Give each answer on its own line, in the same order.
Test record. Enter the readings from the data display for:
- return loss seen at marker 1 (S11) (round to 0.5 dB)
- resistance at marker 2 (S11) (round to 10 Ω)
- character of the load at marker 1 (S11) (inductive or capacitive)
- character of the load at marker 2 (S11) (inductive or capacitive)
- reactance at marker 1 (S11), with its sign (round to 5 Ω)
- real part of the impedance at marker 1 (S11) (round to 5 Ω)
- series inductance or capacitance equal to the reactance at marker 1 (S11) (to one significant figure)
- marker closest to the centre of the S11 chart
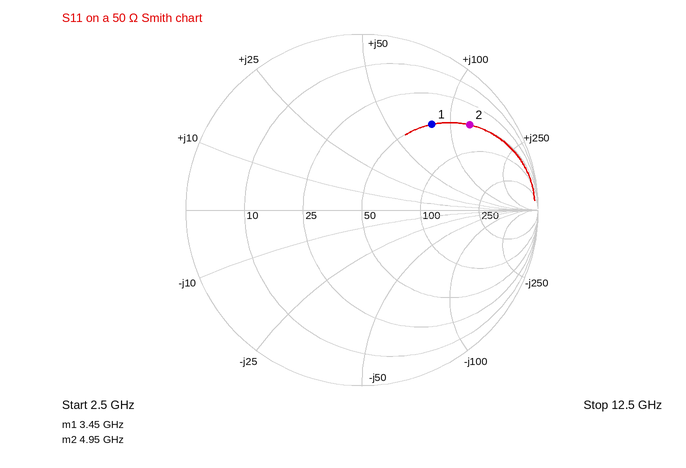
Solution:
4.0 dB
50 Ω
inductive
inductive
+80 Ω
50 Ω
4 nH
marker 1
